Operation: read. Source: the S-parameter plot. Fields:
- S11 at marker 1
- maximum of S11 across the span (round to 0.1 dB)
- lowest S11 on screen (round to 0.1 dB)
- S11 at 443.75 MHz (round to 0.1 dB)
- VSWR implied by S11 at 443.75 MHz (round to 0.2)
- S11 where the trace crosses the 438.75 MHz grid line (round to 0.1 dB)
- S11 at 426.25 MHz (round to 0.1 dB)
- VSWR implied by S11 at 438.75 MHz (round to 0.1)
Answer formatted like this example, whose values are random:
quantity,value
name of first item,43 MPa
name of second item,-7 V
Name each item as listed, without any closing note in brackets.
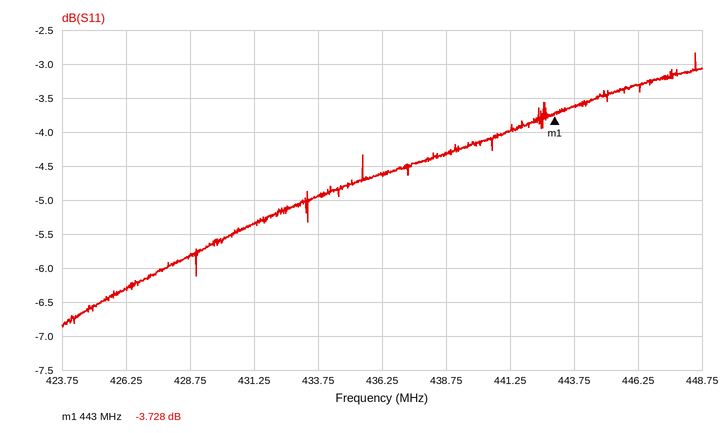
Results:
quantity,value
S11 at marker 1,-3.728 dB
maximum of S11 across the span,-2.8 dB
lowest S11 on screen,-6.9 dB
S11 at 443.75 MHz,-3.6 dB
VSWR implied by S11 at 443.75 MHz,4.8
S11 where the trace crosses the 438.75 MHz grid line,-4.3 dB
S11 at 426.25 MHz,-6.3 dB
VSWR implied by S11 at 438.75 MHz,4.1
